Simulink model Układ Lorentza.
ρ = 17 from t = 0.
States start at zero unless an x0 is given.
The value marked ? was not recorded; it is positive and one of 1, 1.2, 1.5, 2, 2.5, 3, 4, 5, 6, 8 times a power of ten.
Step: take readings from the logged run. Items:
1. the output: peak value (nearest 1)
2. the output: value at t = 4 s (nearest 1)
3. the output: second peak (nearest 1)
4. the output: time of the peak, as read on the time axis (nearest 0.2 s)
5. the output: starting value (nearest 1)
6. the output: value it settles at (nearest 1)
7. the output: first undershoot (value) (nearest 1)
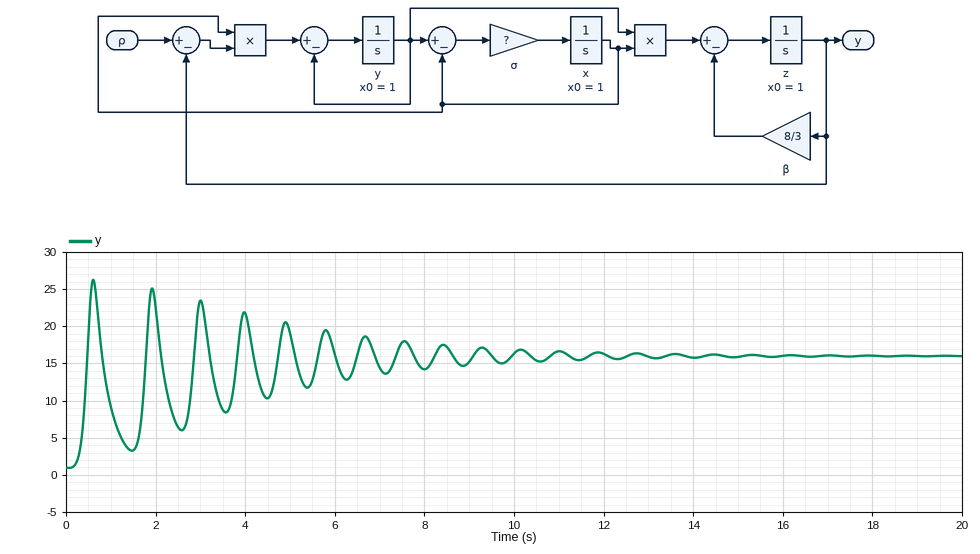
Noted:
26
22
25
0.6 s
1
16
3
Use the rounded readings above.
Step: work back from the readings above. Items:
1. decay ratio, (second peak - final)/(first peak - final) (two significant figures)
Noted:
0.90
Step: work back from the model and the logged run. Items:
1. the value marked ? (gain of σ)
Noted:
5
